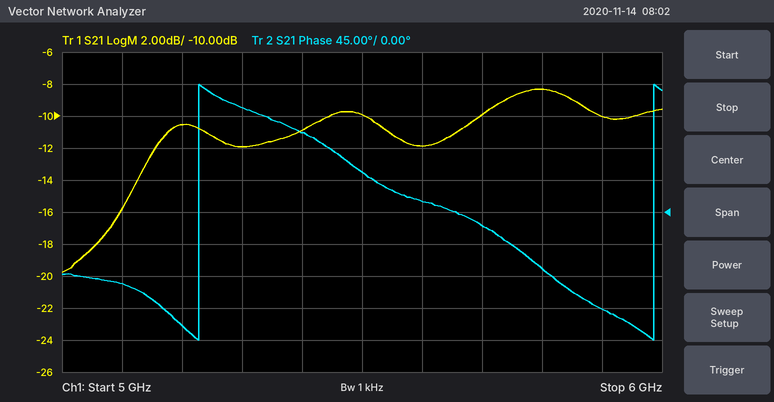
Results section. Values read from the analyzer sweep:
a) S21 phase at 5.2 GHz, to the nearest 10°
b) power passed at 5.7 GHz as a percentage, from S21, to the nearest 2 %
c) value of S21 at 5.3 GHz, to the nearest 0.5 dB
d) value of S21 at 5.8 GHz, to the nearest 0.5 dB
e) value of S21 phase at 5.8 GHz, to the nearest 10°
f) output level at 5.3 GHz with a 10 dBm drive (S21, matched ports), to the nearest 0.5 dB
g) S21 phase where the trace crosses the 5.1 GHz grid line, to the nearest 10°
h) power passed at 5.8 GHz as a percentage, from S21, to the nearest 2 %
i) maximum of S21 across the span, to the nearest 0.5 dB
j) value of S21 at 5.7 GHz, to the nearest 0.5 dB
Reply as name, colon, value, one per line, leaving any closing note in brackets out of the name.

S21 phase at 5.2 GHz, to the nearest 10°: -160°
power passed at 5.7 GHz as a percentage, from S21, to the nearest 2 %: 10 %
value of S21 at 5.3 GHz, to the nearest 0.5 dB: -12.0 dB
value of S21 at 5.8 GHz, to the nearest 0.5 dB: -8.5 dB
value of S21 phase at 5.8 GHz, to the nearest 10°: -80°
output level at 5.3 GHz with a 10 dBm drive (S21, matched ports), to the nearest 0.5 dB: -2.0 dBm
S21 phase where the trace crosses the 5.1 GHz grid line, to the nearest 10°: -100°
power passed at 5.8 GHz as a percentage, from S21, to the nearest 2 %: 14 %
maximum of S21 across the span, to the nearest 0.5 dB: -8.5 dB
value of S21 at 5.7 GHz, to the nearest 0.5 dB: -10.0 dB
